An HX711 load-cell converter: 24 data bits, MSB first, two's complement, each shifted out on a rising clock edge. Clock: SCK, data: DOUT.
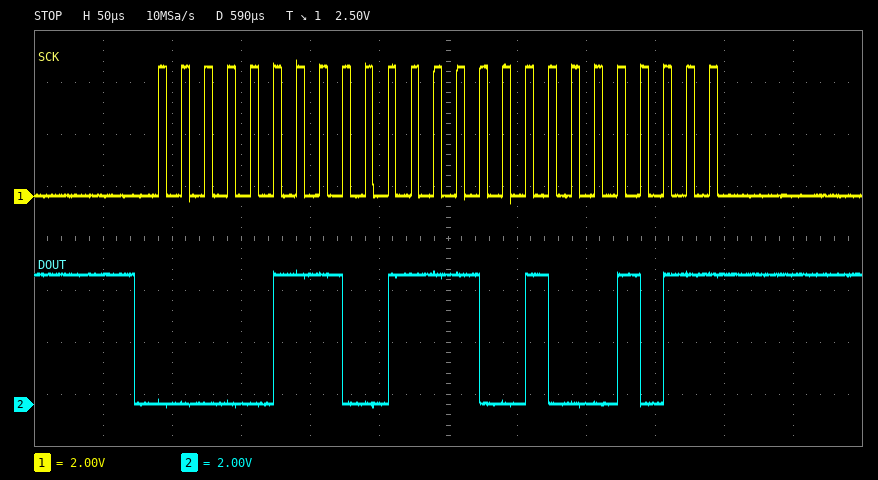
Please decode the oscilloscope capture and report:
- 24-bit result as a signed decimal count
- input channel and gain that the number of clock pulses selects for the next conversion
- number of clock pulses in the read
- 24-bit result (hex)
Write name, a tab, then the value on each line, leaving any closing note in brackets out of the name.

24-bit result as a signed decimal count	474251
input channel and gain that the number of clock pulses selects for the next conversion	channel A, gain 128
number of clock pulses in the read	25
24-bit result	0x073C8B
